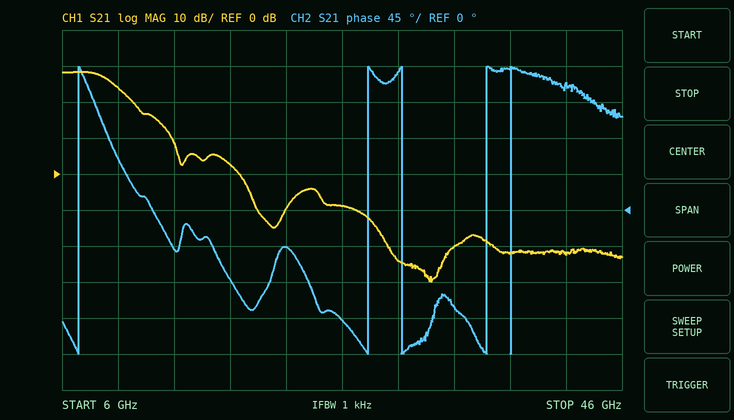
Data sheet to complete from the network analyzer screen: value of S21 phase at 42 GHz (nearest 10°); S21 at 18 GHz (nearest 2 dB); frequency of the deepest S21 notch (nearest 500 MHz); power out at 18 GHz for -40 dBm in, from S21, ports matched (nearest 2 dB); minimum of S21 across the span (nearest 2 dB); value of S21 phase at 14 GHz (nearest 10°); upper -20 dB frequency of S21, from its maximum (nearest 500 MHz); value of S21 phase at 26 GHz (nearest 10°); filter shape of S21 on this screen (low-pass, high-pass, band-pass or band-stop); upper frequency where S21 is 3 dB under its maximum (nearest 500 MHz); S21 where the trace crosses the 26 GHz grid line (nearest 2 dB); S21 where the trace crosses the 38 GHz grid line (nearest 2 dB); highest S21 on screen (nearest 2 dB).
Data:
160°
2 dB
32.5 GHz
-38 dBm
-30 dB
-50°
14.0 GHz
-140°
low-pass
9.5 GHz
-8 dB
-22 dB
28 dB
